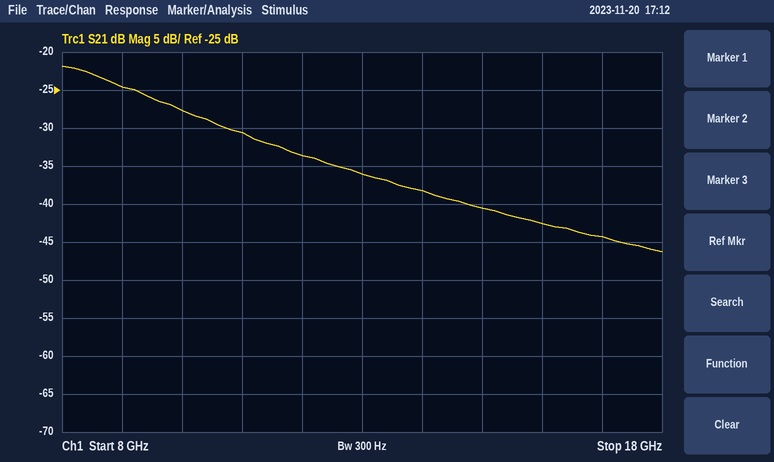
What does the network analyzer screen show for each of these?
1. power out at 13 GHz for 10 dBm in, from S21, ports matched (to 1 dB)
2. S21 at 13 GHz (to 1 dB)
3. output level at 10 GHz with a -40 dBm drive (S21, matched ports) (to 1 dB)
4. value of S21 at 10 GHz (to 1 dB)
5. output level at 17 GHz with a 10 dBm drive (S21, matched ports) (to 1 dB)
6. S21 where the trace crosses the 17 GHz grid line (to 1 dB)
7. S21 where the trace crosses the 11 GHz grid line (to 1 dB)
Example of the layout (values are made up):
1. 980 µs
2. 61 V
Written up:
1. -26 dBm
2. -36 dB
3. -68 dBm
4. -28 dB
5. -34 dBm
6. -44 dB
7. -31 dB
